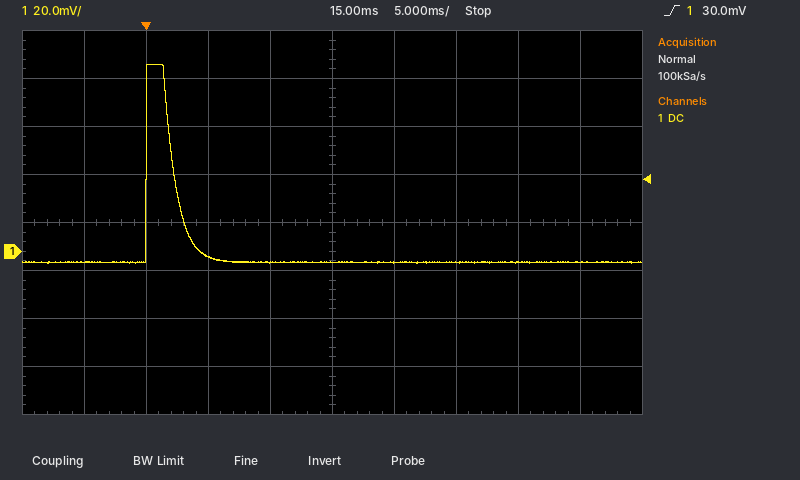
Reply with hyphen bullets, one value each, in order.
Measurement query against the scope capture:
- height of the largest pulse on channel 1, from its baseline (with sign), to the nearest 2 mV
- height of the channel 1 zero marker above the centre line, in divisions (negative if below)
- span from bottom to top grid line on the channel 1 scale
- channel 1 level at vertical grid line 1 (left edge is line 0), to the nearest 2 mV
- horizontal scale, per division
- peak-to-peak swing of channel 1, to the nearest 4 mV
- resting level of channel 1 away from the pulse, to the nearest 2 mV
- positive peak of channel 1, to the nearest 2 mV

- +82 mV
- -0.6 div
- 160 mV
- -4 mV
- 5 ms
- 84 mV
- -4 mV
- 78 mV
